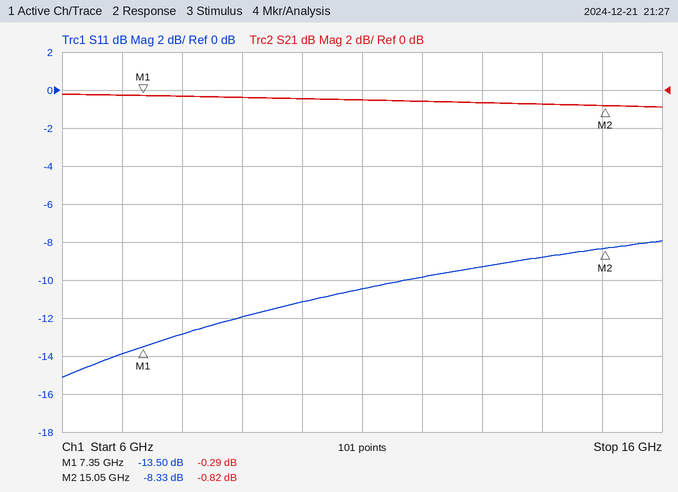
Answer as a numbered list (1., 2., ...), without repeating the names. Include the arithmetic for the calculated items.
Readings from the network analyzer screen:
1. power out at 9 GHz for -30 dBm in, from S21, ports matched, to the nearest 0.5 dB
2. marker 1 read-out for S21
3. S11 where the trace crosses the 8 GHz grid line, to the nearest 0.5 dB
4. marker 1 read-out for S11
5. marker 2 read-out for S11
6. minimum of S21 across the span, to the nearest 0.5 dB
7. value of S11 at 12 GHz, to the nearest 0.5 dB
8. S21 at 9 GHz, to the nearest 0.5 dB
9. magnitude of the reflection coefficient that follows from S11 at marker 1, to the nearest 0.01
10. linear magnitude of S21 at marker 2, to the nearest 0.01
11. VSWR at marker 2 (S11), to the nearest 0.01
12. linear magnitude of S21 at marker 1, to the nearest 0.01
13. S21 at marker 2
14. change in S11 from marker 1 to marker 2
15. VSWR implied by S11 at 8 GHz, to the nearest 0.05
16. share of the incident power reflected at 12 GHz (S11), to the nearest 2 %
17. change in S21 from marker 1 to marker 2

1. -30 dBm + (-0.5 dB) = -30.5 dBm
2. -0.29 dB
3. -13.0 dB
4. -13.50 dB
5. -8.33 dB
6. -1.0 dB
7. -10.0 dB
8. -0.5 dB
9. 10^(-13.5/20) ≈ 0.21
10. 10^(-0.82/20) ≈ 0.91
11. (1 + 0.3833)/(1 − 0.3833) ≈ 2.24
12. 10^(-0.29/20) ≈ 0.97
13. -0.82 dB
14. -8.33 − (-13.5) = 5.17 dB
15. |Γ| = 10^(-13/20) = 0.2239; VSWR = (1 + 0.2239)/(1 − 0.2239) ≈ 1.58, so 1.60 to the nearest 0.05
16. 10^(-10/10) ≈ 10 %
17. -0.82 − (-0.29) = -0.53 dB
